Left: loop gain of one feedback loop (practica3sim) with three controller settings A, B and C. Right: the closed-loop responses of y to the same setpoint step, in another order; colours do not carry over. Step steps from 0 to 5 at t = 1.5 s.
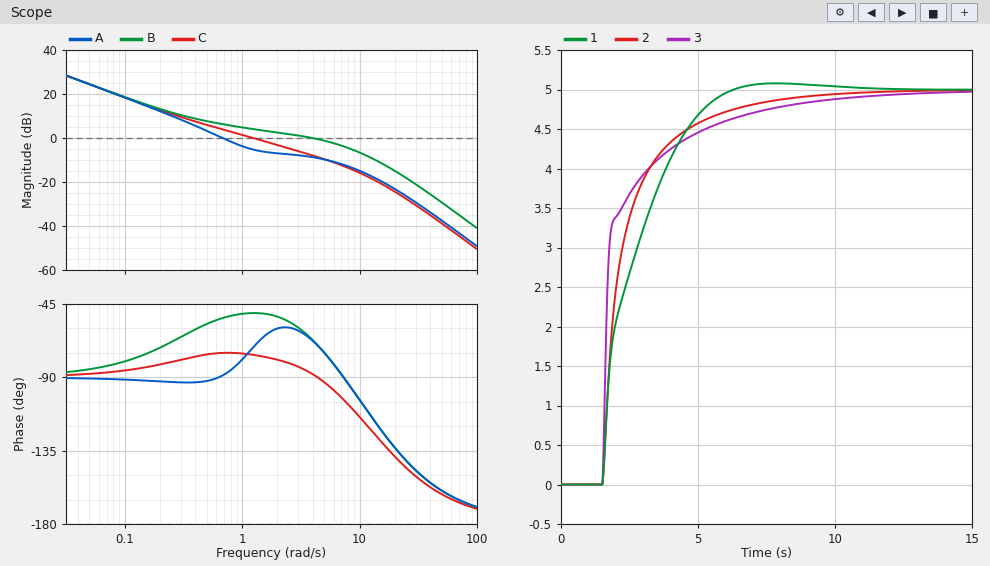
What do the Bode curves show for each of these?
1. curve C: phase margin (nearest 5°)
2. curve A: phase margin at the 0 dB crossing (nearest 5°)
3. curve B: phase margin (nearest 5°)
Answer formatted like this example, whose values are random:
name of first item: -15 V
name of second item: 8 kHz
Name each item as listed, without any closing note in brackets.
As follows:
curve C: phase margin: 105°
curve A: phase margin at the 0 dB crossing: 90°
curve B: phase margin: 115°
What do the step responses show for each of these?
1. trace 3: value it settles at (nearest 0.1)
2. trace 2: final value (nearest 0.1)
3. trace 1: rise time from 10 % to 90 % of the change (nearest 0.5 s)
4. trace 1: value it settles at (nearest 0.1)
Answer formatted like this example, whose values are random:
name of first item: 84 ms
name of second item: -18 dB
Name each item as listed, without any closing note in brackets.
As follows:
trace 3: value it settles at: 5.0
trace 2: final value: 5.0
trace 1: rise time from 10 % to 90 % of the change: 3.0 s
trace 1: value it settles at: 5.0
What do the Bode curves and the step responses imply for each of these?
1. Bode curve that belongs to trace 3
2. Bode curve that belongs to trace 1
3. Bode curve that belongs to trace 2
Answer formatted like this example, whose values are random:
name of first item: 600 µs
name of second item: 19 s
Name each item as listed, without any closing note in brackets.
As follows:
Bode curve that belongs to trace 3: B
Bode curve that belongs to trace 1: A
Bode curve that belongs to trace 2: C
